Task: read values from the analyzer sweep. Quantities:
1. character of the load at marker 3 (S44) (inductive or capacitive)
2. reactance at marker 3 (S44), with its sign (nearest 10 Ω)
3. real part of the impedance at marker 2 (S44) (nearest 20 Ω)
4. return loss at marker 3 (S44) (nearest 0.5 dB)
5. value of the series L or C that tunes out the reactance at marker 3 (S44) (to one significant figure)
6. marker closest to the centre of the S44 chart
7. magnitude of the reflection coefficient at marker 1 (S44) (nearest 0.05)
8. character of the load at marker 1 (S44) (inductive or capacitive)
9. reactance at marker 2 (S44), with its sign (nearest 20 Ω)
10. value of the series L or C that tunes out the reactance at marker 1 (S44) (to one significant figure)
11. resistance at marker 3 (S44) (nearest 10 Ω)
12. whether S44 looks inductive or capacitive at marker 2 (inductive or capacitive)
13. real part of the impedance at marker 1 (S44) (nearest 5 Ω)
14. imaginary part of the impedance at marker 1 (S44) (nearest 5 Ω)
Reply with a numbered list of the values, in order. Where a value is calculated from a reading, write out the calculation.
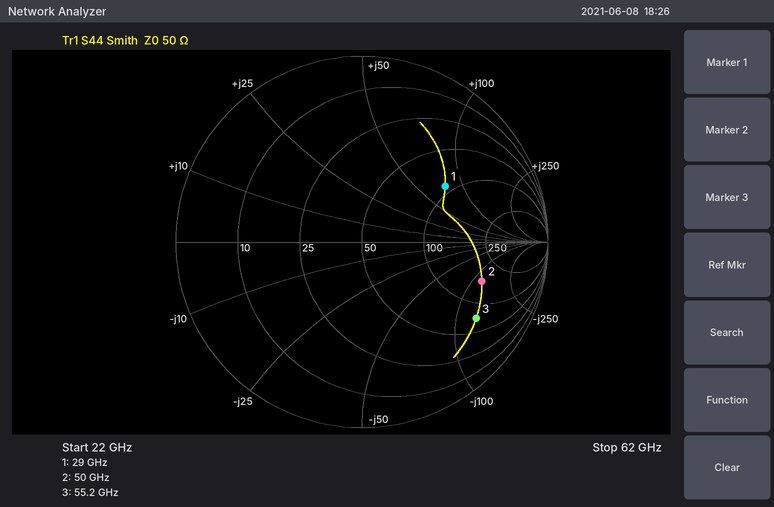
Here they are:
1. capacitive
2. -130 Ω
3. 160 Ω
4. 2.5 dB
5. L = 130 Ω/(2π × 55.2 GHz) ≈ 375 pH, so 400 pH to one significant figure
6. marker 1
7. 0.55
8. inductive
9. -120 Ω
10. C = 1/(2π × 29 GHz × 75 Ω) ≈ 73.2 fF, so 70 fF to one significant figure
11. 70 Ω
12. capacitive
13. 90 Ω
14. +75 Ω
